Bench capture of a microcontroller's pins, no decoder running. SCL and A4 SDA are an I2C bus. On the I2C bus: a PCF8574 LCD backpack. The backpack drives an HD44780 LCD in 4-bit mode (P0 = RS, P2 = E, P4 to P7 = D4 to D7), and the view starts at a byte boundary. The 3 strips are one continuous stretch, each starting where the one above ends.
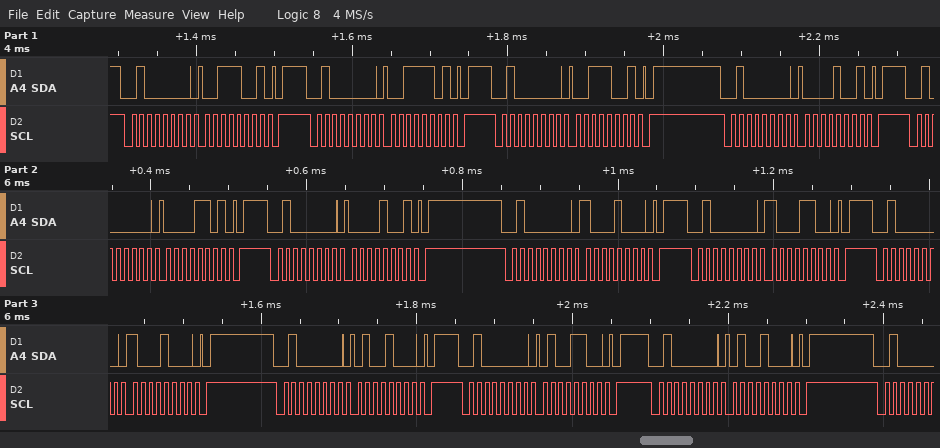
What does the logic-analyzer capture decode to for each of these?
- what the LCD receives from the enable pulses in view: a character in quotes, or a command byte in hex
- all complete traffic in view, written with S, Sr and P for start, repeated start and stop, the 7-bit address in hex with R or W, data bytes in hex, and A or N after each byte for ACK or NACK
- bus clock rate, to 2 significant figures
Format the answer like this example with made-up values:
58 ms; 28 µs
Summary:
'0' 0x84; S 20W A 39 A P S 20W A 3D A P S 20W A 39 A P S 20W A 09 A P S 20W A 0D A P S 20W A 09 A P S 20W A 88 A P S 20W A 8C A P S 20W A 88 A P S 20W A 48 A P S 20W A 4C A P S 20W A 48 A P; 100 kHz
